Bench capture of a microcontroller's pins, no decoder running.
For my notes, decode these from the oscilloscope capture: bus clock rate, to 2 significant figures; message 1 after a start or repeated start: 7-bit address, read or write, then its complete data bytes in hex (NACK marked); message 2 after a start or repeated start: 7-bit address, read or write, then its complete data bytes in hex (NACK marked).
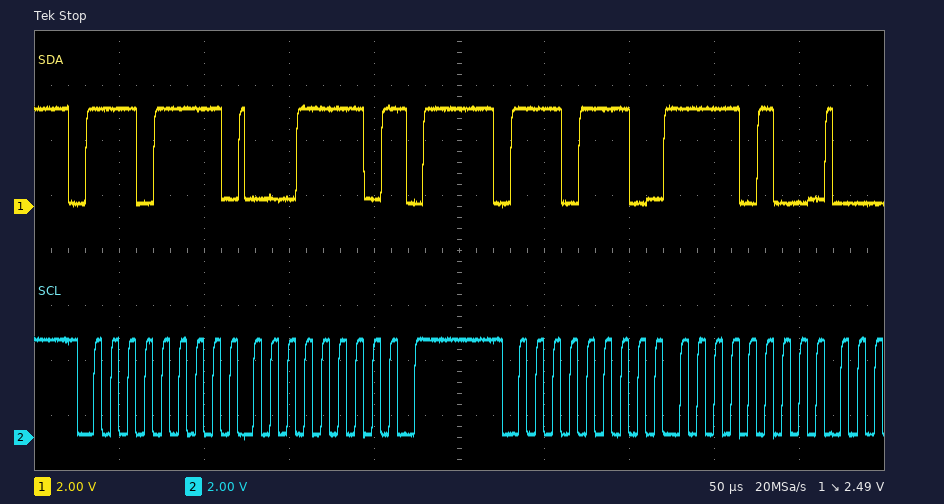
100 kHz
0x77 read: 1E NACK
0x77 write: F4
